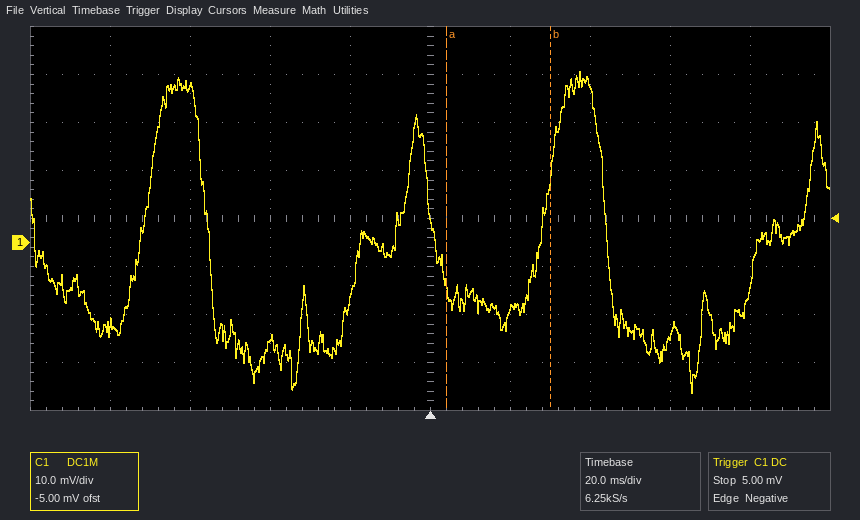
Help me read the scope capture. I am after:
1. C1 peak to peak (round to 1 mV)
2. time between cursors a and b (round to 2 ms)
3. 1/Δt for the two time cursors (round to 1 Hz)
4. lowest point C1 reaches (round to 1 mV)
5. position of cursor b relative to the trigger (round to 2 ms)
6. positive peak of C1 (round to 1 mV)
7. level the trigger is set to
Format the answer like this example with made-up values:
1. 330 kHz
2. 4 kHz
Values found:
1. 67 mV
2. 26 ms
3. 38 Hz
4. -31 mV
5. +30 ms
6. 36 mV
7. 5.00 mV
